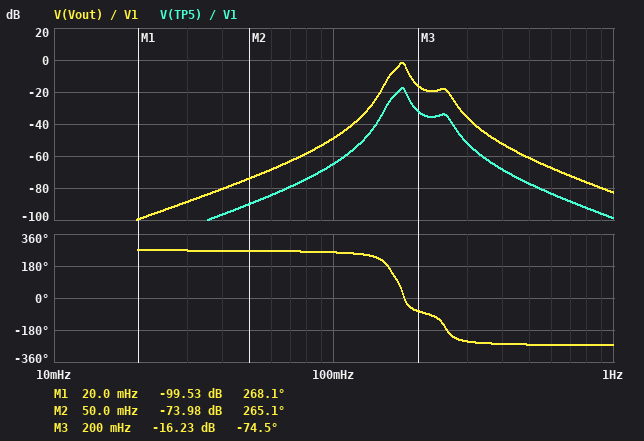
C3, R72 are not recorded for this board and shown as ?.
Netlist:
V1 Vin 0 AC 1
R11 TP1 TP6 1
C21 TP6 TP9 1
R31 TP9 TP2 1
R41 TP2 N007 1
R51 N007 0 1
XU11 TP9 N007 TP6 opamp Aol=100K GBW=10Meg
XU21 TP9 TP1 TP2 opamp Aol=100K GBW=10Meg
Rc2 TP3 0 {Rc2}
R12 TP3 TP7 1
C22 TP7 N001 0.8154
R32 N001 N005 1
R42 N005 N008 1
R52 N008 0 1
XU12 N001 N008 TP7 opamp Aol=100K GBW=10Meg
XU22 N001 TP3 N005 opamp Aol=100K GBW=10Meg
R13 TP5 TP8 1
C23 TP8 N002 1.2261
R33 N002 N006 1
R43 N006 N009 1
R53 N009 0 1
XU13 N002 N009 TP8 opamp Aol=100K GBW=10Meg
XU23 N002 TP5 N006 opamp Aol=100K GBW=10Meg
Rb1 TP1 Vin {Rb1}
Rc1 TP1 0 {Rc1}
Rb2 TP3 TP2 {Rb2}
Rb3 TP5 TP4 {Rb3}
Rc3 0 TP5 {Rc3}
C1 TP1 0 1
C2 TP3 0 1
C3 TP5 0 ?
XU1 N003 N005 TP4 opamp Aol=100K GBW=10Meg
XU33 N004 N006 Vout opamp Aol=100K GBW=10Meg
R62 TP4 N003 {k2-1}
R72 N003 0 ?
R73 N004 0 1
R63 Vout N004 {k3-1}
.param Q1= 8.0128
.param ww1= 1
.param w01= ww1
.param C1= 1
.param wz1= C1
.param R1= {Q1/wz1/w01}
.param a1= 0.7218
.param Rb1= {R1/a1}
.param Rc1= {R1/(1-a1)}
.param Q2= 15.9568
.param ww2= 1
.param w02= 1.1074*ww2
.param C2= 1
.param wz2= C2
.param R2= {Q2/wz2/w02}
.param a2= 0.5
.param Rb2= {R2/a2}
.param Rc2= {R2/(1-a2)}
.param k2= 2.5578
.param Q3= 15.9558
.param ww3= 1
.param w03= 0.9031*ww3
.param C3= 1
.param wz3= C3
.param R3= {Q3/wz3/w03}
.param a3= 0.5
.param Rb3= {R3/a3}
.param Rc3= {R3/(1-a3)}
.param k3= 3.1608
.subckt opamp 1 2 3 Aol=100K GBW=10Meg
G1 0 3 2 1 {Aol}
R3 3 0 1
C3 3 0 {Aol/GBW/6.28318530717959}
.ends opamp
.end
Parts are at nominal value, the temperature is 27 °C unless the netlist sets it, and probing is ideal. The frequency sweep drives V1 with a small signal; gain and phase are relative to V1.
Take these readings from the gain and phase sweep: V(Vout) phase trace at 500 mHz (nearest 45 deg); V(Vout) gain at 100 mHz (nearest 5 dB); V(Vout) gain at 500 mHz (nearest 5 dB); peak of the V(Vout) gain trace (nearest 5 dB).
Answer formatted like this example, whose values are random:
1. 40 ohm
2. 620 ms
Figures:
1. -270 deg
2. -50 dB
3. -60 dB
4. 0 dB
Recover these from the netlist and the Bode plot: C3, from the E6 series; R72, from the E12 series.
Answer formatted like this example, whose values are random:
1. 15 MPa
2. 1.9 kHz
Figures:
1. 330 mF
2. 1.2 Ω
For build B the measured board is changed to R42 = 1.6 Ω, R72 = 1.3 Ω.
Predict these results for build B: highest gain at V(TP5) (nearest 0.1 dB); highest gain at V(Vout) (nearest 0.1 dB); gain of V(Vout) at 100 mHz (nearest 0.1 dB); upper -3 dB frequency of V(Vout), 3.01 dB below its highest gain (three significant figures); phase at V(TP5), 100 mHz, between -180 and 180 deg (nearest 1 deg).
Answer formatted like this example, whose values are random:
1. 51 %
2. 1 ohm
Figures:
1. -16.0 dB
2. 0 dB
3. -52.3 dB
4. 230 mHz
5. -102 deg
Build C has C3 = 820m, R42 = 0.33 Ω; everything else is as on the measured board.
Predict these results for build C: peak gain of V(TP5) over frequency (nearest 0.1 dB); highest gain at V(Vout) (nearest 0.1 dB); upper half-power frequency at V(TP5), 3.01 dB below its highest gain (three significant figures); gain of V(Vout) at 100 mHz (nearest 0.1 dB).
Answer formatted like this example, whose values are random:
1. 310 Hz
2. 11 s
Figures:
1. -17.8 dB
2. -1.8 dB
3. 163 mHz
4. -24.0 dB
